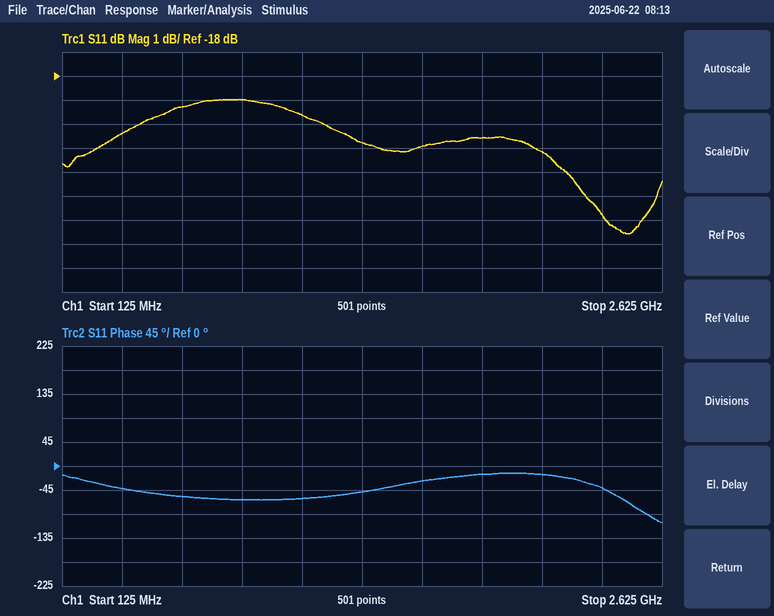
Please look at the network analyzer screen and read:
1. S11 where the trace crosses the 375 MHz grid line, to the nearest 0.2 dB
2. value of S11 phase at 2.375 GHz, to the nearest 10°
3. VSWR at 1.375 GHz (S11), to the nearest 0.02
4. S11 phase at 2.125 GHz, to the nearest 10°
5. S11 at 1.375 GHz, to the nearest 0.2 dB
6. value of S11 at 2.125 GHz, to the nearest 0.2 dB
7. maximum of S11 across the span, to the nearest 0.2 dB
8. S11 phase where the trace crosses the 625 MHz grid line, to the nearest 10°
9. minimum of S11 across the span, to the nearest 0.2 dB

-20.4 dB
-40°
1.20
-20°
-20.8 dB
-21.2 dB
-19.0 dB
-60°
-24.6 dB
